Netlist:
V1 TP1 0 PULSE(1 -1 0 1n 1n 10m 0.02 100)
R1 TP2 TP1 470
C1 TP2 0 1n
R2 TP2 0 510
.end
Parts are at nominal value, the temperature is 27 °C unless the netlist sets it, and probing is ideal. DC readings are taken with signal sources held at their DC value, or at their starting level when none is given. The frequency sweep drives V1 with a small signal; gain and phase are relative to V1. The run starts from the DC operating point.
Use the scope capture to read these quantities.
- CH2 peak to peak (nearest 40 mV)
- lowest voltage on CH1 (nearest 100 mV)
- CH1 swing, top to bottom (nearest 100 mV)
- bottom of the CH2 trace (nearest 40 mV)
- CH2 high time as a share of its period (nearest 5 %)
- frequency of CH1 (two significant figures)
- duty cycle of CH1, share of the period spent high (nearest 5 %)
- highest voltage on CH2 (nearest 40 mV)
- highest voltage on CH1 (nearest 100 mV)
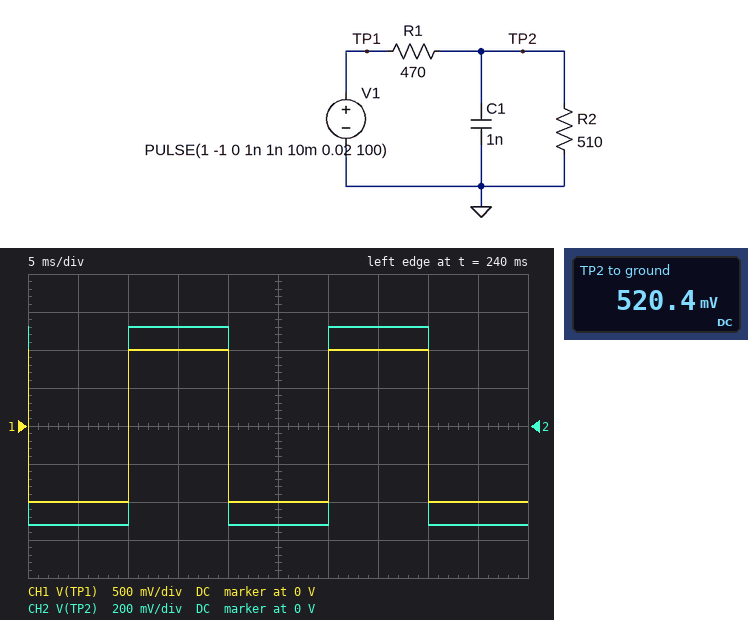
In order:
1.04 V
-1.0 V
2.0 V
-520 mV
50 %
50 Hz
50 %
520 mV
1.0 V
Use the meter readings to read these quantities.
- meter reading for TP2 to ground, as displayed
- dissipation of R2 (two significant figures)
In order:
520.4 mV
530 µW
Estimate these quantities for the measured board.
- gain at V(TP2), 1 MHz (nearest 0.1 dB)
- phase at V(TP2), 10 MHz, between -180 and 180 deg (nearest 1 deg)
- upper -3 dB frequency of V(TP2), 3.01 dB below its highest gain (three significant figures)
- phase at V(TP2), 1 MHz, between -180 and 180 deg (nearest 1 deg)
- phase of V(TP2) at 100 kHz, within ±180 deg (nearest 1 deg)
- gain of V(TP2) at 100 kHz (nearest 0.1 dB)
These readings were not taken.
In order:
-10.9 dB
-86 deg
651 kHz
-57 deg
-9 deg
-5.8 dB
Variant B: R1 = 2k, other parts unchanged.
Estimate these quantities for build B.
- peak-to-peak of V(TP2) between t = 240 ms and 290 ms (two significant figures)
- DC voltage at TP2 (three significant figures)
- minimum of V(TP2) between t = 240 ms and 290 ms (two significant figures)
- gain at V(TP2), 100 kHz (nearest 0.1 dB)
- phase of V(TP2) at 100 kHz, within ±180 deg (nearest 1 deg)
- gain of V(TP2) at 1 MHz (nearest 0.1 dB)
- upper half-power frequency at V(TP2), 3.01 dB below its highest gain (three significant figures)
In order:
410 mV
203 mV
-200 mV
-14.1 dB
-14 deg
-22.6 dB
392 kHz
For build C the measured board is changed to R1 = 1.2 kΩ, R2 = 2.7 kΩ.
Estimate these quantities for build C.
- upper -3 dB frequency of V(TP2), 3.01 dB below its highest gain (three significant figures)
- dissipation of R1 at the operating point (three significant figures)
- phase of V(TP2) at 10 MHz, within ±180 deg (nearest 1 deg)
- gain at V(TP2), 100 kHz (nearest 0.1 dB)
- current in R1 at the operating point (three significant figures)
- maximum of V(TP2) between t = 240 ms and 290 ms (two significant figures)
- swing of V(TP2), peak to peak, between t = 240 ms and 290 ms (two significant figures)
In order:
192 kHz
78.9 µW
-89 deg
-4.2 dB
256 µA
690 mV
1.4 V
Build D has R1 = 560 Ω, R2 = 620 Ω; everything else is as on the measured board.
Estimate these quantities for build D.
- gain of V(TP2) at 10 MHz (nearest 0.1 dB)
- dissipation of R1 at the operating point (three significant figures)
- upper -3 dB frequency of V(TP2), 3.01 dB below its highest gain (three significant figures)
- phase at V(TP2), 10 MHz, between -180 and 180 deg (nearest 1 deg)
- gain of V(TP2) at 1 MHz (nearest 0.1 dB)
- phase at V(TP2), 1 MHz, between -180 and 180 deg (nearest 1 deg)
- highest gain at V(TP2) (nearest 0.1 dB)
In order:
-30.9 dB
402 µW
541 kHz
-87 deg
-12.0 dB
-62 deg
-5.6 dB
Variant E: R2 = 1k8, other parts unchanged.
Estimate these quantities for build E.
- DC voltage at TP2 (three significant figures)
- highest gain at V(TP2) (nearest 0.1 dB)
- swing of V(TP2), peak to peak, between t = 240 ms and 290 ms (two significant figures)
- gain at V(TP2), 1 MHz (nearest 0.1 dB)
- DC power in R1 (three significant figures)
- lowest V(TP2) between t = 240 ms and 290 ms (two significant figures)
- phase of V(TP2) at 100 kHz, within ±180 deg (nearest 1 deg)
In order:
793 mV
-2.0 dB
1.6 V
-10.1 dB
91.2 µW
-790 mV
-13 deg
